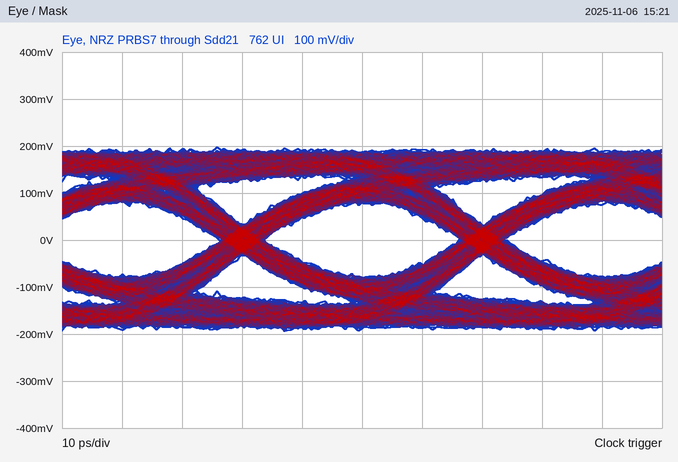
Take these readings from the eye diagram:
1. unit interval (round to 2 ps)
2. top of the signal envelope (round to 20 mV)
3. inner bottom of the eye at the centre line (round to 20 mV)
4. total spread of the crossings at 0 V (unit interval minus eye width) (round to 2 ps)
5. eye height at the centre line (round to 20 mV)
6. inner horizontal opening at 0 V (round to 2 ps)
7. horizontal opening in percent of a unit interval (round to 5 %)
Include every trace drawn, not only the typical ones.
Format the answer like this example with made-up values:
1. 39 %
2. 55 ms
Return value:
1. 40 ps
2. 200 mV
3. -80 mV
4. 8 ps
5. 160 mV
6. 32 ps
7. 80 %
